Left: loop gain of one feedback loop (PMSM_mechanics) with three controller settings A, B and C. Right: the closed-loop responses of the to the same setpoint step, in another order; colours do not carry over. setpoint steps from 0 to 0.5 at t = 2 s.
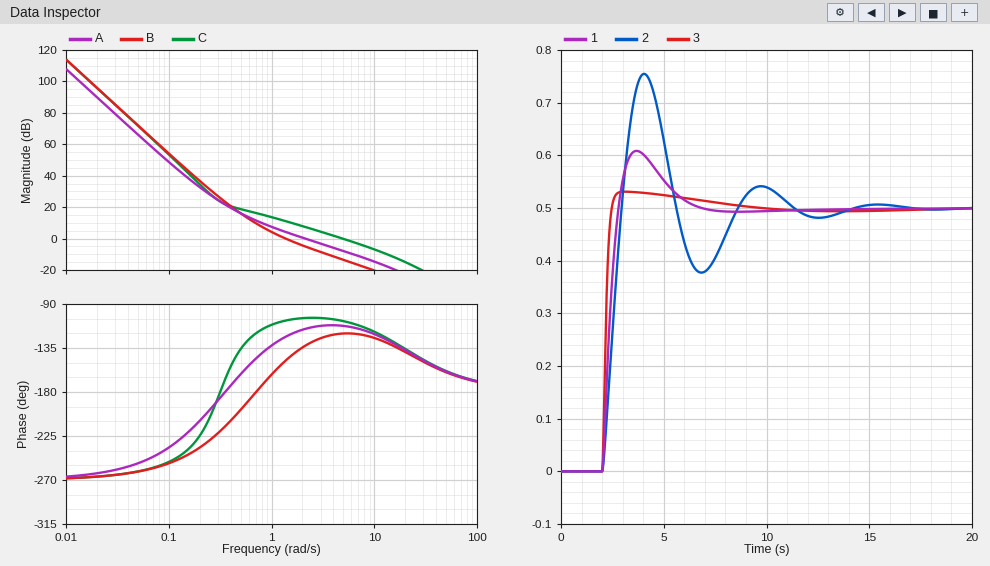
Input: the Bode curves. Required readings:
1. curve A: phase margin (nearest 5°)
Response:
65°
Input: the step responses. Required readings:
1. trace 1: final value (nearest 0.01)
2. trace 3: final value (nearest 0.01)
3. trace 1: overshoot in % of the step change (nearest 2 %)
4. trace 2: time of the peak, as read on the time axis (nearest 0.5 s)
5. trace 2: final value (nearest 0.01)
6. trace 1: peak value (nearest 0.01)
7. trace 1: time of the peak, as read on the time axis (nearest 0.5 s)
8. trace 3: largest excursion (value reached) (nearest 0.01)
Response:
0.50
0.50
22 %
4.0 s
0.50
0.61
3.5 s
0.53
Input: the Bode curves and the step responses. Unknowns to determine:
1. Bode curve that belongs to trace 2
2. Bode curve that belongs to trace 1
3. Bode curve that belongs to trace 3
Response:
B
A
C
